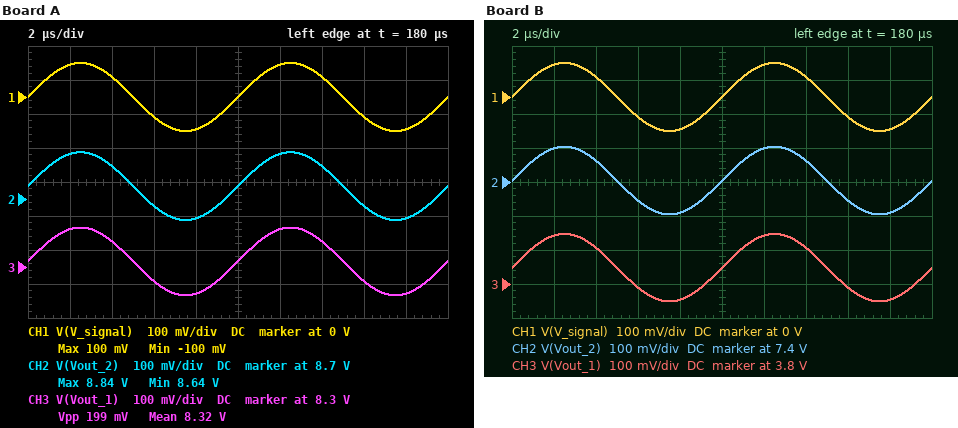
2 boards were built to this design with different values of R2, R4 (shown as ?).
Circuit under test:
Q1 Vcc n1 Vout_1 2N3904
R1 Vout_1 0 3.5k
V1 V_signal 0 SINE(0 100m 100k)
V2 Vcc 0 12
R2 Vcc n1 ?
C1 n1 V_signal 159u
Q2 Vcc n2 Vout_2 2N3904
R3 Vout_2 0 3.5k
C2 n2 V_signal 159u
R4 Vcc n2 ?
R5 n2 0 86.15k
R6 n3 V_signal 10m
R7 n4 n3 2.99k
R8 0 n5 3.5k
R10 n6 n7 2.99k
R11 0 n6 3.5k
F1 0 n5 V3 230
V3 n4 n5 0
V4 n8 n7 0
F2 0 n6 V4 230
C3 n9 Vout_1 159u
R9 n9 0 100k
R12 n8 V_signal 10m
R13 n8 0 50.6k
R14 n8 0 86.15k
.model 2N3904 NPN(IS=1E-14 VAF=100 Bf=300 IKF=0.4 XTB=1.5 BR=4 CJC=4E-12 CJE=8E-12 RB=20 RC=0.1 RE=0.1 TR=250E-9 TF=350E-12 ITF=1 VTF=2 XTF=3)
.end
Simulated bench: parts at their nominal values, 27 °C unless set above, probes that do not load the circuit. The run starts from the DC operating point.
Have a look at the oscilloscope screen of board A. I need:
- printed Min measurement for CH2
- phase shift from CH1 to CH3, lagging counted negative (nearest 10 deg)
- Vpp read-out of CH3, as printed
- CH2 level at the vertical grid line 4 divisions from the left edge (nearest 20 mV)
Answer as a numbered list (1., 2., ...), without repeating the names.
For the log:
1. 8.64 V
2. 0 deg
3. 199 mV
4. 8.64 V
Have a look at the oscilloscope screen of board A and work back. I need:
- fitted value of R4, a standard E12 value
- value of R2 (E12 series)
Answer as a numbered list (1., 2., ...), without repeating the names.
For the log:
1. 22 kΩ
2. 390 kΩ
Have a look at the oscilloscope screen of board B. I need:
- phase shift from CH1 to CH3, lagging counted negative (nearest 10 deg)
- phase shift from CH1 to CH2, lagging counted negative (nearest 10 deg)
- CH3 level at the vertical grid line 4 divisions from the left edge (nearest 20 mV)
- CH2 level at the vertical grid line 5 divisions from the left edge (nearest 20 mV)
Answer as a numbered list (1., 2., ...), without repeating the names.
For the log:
1. 0 deg
2. 0 deg
3. 3.76 V
4. 7.40 V
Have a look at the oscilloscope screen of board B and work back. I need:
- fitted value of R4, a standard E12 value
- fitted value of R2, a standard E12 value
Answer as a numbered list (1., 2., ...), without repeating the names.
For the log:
1. 39 kΩ
2. 2.2 MΩ
